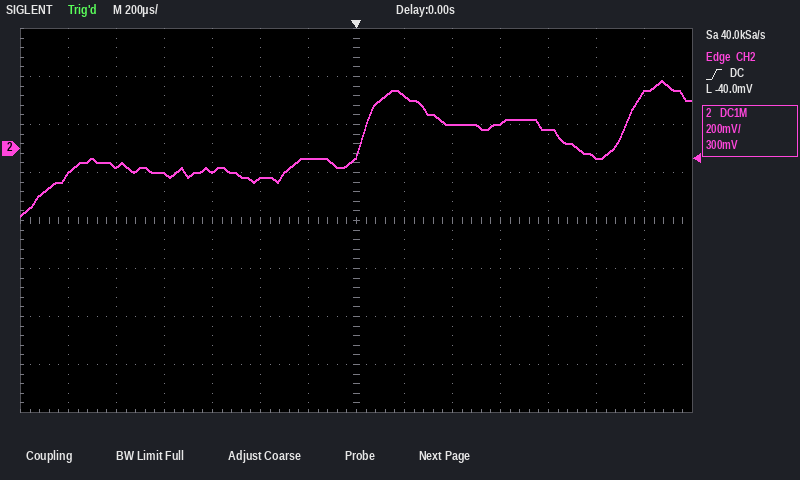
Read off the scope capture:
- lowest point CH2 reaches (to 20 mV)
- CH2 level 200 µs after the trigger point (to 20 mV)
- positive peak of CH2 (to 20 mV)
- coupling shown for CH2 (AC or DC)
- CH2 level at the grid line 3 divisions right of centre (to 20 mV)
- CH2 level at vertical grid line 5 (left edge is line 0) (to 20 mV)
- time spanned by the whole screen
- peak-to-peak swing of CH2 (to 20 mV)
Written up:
-280 mV
220 mV
280 mV
DC
100 mV
-120 mV
2.8 ms
560 mV
